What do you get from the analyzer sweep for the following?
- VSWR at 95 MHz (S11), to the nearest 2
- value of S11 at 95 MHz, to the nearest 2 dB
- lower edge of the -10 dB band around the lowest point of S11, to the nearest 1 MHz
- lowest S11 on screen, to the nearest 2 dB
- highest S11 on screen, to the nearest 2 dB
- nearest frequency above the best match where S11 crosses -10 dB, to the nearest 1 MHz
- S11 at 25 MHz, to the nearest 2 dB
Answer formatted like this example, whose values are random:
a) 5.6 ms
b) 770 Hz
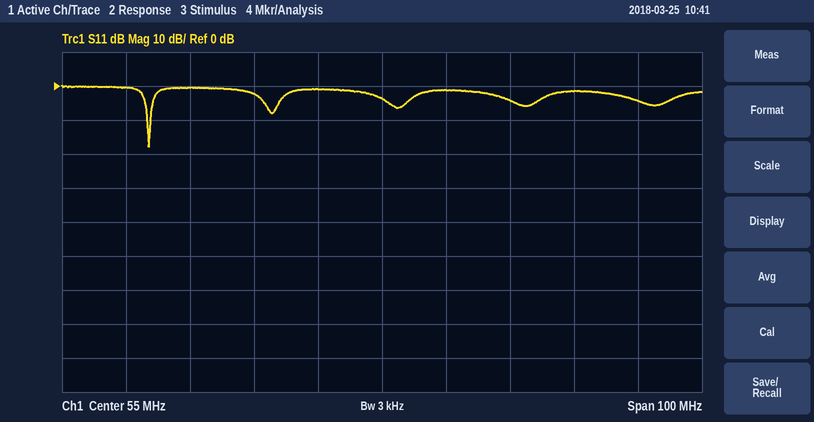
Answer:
a) 4
b) -4 dB
c) 18 MHz
d) -18 dB
e) 0 dB
f) 19 MHz
g) 0 dB
